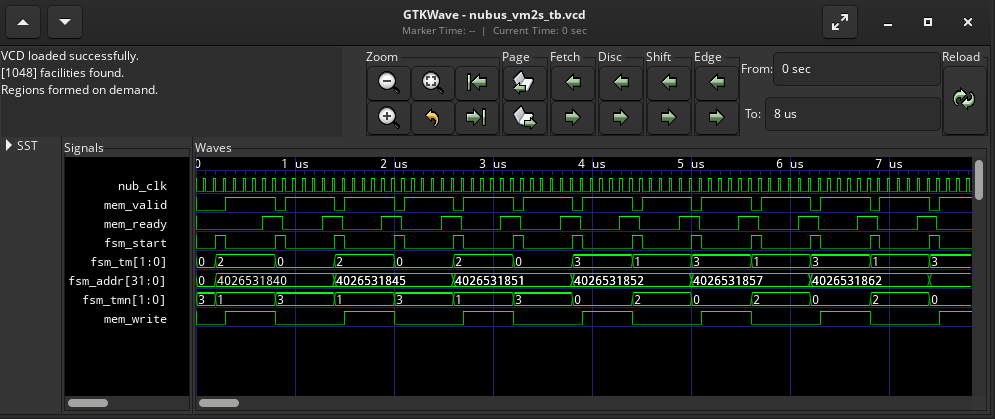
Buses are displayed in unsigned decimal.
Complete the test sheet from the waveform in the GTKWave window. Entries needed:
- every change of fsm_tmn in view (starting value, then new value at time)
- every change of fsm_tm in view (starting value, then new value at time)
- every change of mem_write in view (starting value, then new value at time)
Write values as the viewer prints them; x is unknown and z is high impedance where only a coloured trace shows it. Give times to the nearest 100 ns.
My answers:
3, 1 at 200 ns, 3 at 800 ns, 1 at 1400 ns, 3 at 2000 ns, 1 at 2600 ns, 3 at 3200 ns, 0 at 3800 ns, 2 at 4400 ns, 0 at 5000 ns, 2 at 5600 ns, 0 at 6200 ns, 2 at 6800 ns, 0 at 7400 ns
0, 2 at 200 ns, 0 at 800 ns, 2 at 1400 ns, 0 at 2000 ns, 2 at 2600 ns, 0 at 3200 ns, 3 at 3800 ns, 1 at 4400 ns, 3 at 5000 ns, 1 at 5600 ns, 3 at 6200 ns, 1 at 6800 ns, 3 at 7400 ns
0, 1 at 300 ns, 0 at 800 ns, 1 at 1500 ns, 0 at 2000 ns, 1 at 2700 ns, 0 at 3200 ns, 1 at 3900 ns, 0 at 4400 ns, 1 at 5100 ns, 0 at 5600 ns, 1 at 6300 ns, 0 at 6800 ns, 1 at 7500 ns
